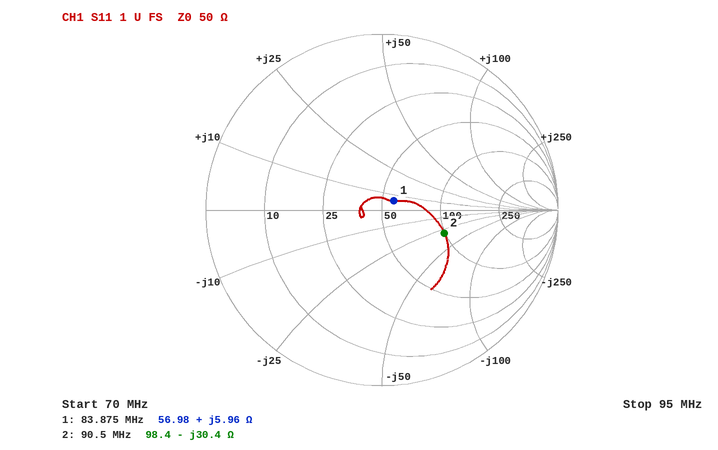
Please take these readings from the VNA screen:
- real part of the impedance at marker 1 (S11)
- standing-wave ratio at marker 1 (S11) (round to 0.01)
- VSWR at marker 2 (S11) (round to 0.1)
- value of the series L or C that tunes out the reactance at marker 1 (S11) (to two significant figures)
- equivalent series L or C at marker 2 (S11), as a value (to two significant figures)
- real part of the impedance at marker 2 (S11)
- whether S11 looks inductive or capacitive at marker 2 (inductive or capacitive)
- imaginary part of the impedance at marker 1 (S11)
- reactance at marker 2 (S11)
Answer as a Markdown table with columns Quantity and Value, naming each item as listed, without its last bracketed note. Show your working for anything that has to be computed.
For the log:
| Quantity | Value |
|---|---|
| real part of the impedance at marker 1 | 56.98 Ω |
| standing-wave ratio at marker 1 (S11) | 1.19 |
| VSWR at marker 2 (S11) | 2.2 |
| value of the series L or C that tunes out the reactance at marker 1 (S11) | C = 1/(2π × 83.875 MHz × 5.96 Ω) ≈ 318 pF, so 320 pF to two significant figures |
| equivalent series L or C at marker 2 (S11), as a value | C = 1/(2π × 90.5 MHz × 30.4 Ω) ≈ 58 pF |
| real part of the impedance at marker 2 | 98.4 Ω |
| whether S11 looks inductive or capacitive at marker 2 | capacitive |
| imaginary part of the impedance at marker 1 | +5.96 Ω |
| reactance at marker 2 | -30.4 Ω |
